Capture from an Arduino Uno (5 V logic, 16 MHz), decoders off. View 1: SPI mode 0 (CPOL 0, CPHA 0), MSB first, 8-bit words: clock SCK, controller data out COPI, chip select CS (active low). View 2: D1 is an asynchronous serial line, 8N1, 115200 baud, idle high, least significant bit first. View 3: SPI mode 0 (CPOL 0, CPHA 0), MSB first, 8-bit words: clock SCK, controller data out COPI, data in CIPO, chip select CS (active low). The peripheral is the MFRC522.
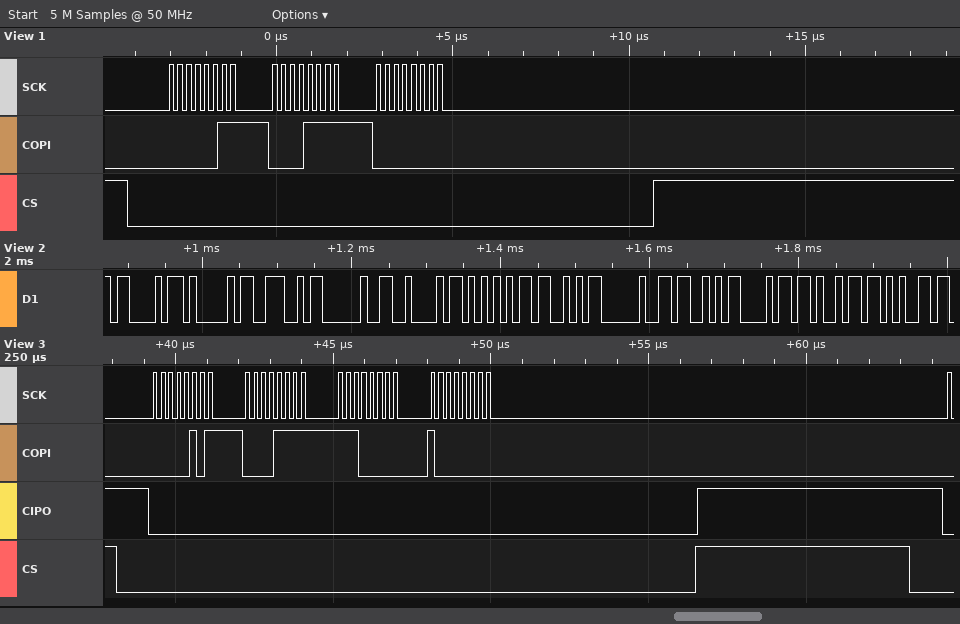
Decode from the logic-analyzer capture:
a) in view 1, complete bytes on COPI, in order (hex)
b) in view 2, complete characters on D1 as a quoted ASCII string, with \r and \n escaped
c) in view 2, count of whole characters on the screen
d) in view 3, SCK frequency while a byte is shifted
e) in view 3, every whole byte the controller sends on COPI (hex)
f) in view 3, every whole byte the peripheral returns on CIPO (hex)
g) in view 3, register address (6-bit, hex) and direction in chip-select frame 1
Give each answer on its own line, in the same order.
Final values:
03 0F 00
"CAN BUS Shie"
12
4 MHz
0x05 0x0F 0xE0 0x80
0x00 0x00 0x00 0x00
0x02 write
